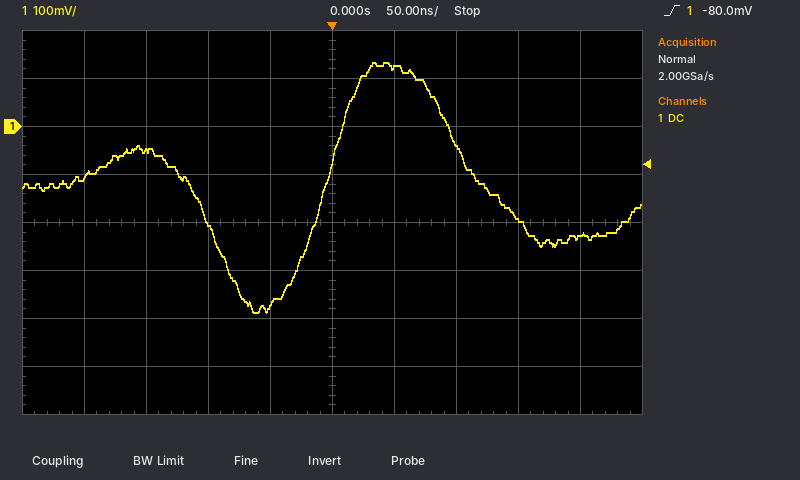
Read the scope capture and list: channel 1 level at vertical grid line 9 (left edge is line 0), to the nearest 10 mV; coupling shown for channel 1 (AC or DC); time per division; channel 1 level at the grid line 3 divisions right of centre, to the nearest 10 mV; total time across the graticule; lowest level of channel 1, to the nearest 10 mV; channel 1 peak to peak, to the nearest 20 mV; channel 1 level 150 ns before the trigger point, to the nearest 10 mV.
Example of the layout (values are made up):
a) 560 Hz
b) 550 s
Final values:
a) -230 mV
b) DC
c) 50 ns
d) -190 mV
e) 500 ns
f) -390 mV
g) 520 mV
h) -50 mV
